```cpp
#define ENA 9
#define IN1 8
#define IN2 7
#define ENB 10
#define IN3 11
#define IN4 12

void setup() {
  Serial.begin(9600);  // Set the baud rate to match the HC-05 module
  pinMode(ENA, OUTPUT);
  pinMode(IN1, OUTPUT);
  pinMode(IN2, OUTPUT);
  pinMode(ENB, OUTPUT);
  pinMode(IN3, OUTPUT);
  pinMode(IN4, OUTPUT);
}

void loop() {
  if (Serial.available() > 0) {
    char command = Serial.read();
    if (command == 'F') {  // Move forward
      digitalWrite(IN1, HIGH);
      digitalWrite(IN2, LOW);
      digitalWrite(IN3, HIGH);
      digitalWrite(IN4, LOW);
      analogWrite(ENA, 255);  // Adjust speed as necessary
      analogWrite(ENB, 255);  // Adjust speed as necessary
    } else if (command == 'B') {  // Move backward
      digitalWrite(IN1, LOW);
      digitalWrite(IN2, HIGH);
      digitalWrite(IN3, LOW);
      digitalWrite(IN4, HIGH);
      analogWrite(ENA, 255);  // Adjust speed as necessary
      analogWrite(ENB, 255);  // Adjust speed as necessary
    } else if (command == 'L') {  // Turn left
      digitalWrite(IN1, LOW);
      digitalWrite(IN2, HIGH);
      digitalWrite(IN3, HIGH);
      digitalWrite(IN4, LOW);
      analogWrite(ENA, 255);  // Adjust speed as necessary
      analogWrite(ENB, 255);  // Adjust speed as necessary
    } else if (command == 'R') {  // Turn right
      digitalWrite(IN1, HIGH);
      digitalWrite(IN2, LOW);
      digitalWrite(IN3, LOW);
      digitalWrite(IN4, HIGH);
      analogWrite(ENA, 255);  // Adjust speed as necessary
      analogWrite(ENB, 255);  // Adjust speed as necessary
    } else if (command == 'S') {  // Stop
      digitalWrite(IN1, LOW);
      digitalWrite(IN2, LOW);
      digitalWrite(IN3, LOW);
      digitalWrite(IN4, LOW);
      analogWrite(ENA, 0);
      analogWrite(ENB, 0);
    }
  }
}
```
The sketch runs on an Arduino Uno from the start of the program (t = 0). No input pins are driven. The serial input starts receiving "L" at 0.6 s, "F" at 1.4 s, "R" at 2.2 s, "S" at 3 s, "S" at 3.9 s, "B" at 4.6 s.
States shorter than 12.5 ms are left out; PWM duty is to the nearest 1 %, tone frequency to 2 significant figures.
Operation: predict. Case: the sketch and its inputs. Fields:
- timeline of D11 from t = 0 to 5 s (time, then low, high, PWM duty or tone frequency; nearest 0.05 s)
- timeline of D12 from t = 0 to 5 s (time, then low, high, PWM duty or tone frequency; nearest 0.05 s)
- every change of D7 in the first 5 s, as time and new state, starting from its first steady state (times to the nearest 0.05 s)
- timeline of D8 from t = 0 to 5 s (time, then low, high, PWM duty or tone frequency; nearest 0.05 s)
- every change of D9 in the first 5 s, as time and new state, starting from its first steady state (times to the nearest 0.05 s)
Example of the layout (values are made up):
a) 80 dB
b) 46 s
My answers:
a) 0 s low; 0.6 s high; 2.2 s low
b) 0 s low; 2.2 s high; 3 s low; 4.6 s high
c) 0 s low; 0.6 s high; 1.4 s low; 4.6 s high
d) 0 s low; 1.4 s high; 3 s low
e) 0 s low; 0.6 s high; 3 s low; 4.6 s high
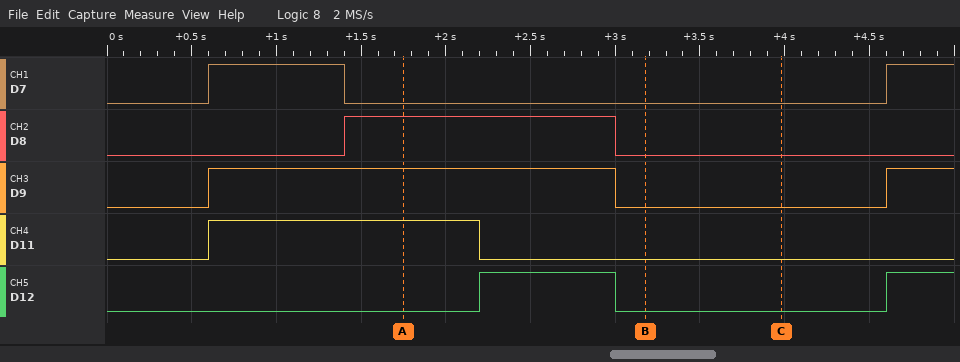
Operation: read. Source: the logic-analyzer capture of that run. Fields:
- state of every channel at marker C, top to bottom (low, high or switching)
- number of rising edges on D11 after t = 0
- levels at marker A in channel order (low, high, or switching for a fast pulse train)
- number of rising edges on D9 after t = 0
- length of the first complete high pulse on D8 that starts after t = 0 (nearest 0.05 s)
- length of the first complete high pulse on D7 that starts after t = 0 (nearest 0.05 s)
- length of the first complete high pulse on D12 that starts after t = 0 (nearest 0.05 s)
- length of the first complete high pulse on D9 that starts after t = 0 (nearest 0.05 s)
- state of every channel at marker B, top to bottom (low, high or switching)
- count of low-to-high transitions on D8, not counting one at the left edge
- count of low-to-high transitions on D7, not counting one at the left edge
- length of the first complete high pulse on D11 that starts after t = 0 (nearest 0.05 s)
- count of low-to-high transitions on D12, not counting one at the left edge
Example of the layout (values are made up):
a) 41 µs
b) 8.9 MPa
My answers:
a) D7 low, D8 low, D9 low, D11 low, D12 low
b) 1
c) D7 low, D8 high, D9 high, D11 high, D12 low
d) 2
e) 1.60 s
f) 0.80 s
g) 0.80 s
h) 2.40 s
i) D7 low, D8 low, D9 low, D11 low, D12 low
j) 1
k) 2
l) 1.60 s
m) 2
